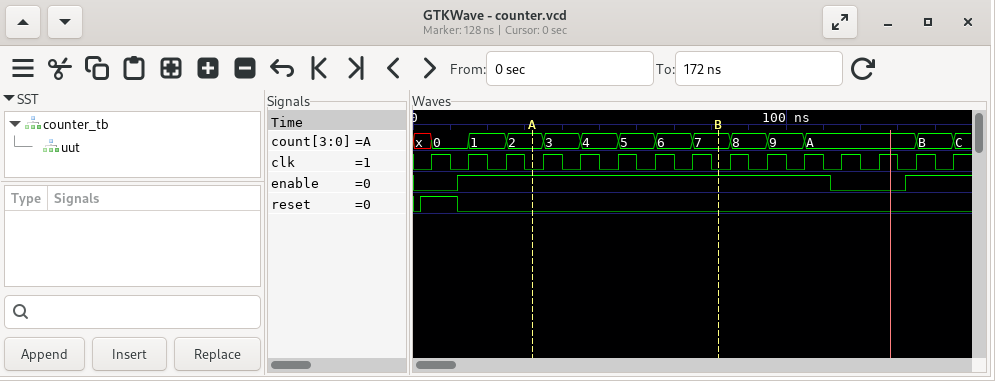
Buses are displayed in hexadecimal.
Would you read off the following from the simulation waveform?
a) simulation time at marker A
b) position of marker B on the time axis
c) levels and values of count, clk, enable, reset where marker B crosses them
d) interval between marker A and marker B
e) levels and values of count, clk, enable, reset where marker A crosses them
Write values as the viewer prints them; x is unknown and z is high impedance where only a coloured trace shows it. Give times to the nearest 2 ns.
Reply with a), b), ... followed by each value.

a) 32 ns
b) 82 ns
c) count=7, clk=0, enable=1, reset=0
d) 50 ns
e) count=2, clk=0, enable=1, reset=0
